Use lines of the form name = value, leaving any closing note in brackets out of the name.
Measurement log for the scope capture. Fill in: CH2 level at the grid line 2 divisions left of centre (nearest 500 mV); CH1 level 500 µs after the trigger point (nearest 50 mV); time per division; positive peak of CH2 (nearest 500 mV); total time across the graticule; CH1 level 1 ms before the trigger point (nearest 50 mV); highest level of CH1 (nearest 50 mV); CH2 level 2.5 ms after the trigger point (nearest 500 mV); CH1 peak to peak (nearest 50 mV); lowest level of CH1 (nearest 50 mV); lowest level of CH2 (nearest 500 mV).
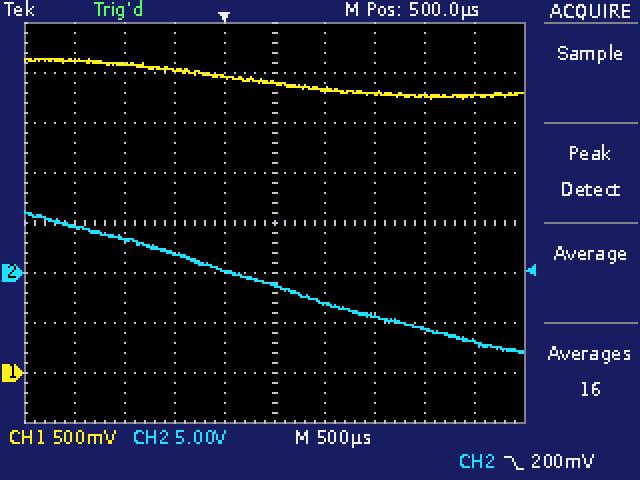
CH2 level at the grid line 2 divisions left of centre = 2.0 V
CH1 level 500 µs after the trigger point = 2.90 V
time per division = 500 µs
positive peak of CH2 = 6.0 V
total time across the graticule = 5 ms
CH1 level 1 ms before the trigger point = 3.10 V
highest level of CH1 = 3.15 V
CH2 level 2.5 ms after the trigger point = -7.0 V
CH1 peak to peak = 400 mV
lowest level of CH1 = 2.75 V
lowest level of CH2 = -8.0 V
